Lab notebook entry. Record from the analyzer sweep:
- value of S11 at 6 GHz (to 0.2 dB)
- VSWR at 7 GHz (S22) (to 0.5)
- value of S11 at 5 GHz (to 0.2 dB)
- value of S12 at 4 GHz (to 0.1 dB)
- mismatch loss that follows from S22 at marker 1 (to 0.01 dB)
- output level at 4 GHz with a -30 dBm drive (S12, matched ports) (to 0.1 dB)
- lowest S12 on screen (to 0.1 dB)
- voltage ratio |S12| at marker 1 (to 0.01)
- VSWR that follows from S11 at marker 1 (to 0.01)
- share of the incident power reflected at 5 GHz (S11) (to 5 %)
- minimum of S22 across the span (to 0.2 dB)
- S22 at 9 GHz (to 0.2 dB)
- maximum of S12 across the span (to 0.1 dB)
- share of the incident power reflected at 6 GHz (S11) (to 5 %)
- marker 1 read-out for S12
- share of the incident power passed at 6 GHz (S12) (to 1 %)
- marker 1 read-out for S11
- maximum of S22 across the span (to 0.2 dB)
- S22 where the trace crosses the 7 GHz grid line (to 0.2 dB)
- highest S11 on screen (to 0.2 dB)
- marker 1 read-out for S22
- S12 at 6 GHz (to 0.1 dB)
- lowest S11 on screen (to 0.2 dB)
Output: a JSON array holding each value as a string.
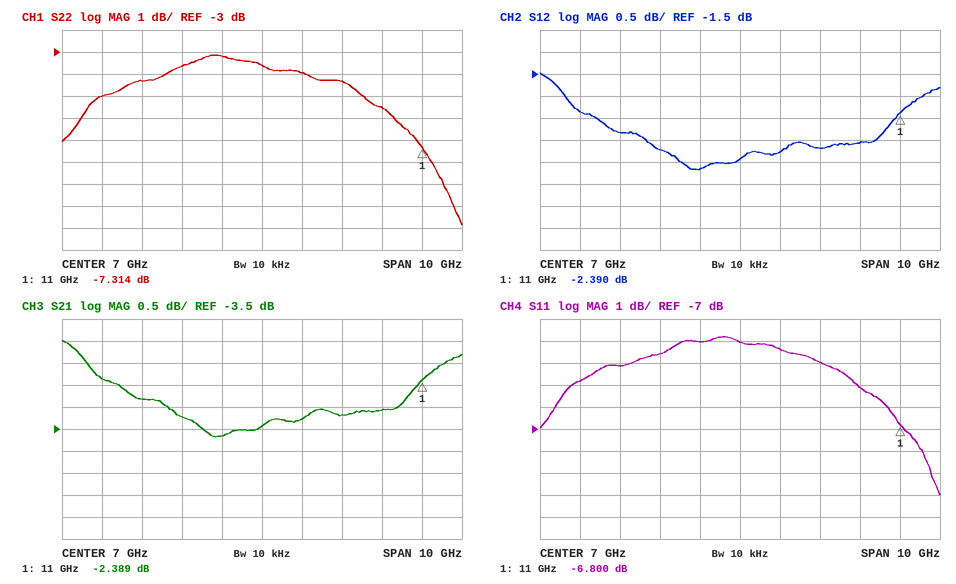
["-3.0 dB", "5.0", "-3.6 dB", "-2.8 dB", "0.89 dB", "-32.8 dBm", "-3.7 dB", "0.76", "2.68", "45 %", "-10.8 dB", "-4.4 dB", "-1.5 dB", "50 %", "-2.390 dB", "43 %", "-6.800 dB", "-3.2 dB", "-3.6 dB", "-2.8 dB", "-7.314 dB", "-3.7 dB", "-10.0 dB"]
